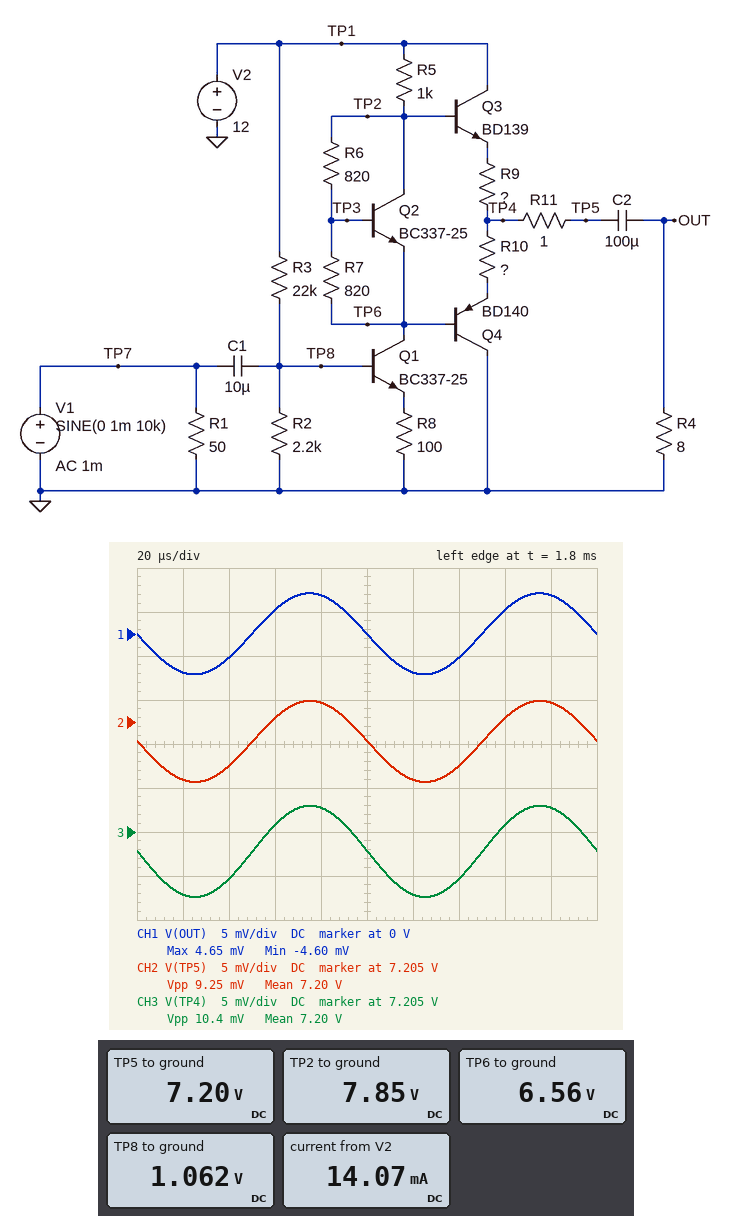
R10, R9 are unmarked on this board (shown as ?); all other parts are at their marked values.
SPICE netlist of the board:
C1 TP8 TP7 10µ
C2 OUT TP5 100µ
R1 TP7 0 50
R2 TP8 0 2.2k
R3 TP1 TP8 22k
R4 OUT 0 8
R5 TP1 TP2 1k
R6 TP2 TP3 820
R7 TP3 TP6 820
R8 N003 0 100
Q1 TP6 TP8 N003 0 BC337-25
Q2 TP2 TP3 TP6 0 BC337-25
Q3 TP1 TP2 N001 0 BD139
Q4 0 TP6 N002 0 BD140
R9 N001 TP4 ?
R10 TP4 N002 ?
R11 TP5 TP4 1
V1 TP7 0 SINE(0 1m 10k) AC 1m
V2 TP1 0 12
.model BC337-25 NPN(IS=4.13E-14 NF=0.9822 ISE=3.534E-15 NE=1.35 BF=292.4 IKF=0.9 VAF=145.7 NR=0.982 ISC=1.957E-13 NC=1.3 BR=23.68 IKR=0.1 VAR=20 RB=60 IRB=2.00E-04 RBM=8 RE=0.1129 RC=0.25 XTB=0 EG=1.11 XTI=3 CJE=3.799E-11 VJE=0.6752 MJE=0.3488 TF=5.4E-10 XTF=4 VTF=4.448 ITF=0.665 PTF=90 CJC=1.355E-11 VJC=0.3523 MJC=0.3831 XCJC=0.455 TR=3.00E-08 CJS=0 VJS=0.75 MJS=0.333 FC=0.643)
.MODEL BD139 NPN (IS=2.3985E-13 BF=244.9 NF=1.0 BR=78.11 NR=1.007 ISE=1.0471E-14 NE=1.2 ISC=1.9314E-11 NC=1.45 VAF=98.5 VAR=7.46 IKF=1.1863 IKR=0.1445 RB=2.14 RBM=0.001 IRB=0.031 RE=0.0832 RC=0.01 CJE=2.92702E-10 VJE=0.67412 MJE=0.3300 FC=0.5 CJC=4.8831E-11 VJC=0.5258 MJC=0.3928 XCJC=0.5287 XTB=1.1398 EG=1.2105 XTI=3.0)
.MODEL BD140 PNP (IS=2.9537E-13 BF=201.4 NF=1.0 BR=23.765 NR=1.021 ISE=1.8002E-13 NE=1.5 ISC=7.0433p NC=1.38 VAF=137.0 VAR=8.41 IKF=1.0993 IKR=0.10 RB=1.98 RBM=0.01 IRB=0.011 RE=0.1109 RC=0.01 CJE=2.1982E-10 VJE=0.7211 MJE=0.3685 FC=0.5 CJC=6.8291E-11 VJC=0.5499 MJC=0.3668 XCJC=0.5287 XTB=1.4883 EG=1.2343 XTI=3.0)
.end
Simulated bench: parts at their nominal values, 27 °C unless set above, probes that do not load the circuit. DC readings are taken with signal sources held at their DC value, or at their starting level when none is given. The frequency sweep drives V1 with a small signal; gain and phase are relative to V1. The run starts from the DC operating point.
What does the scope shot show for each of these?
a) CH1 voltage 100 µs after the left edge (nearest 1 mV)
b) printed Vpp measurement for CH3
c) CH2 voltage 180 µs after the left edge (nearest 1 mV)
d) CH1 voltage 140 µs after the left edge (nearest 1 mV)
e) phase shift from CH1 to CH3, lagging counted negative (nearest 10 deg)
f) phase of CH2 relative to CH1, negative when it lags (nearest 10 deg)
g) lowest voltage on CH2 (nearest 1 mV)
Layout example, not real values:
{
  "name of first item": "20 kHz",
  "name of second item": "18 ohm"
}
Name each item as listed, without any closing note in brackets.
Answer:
{
  "CH1 voltage 100 µs after the left edge": "0 V",
  "printed Vpp measurement for CH3": "10.4 mV",
  "CH2 voltage 180 µs after the left edge": "7.207 V",
  "CH1 voltage 140 µs after the left edge": "-3 mV",
  "phase shift from CH1 to CH3, lagging counted negative": "0 deg",
  "phase of CH2 relative to CH1, negative when it lags": "0 deg",
  "lowest voltage on CH2": "7.198 V"
}
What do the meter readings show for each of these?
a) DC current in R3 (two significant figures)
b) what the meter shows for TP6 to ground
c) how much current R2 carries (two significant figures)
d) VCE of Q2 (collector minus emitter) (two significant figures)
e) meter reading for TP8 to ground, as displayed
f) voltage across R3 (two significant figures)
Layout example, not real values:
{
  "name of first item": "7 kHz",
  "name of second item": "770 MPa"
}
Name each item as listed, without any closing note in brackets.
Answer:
{
  "DC current in R3": "500 µA",
  "what the meter shows for TP6 to ground": "6.56 V",
  "how much current R2 carries": "480 µA",
  "VCE of Q2 (collector minus emitter)": "1.3 V",
  "meter reading for TP8 to ground, as displayed": "1.062 V",
  "voltage across R3": "11 V"
}
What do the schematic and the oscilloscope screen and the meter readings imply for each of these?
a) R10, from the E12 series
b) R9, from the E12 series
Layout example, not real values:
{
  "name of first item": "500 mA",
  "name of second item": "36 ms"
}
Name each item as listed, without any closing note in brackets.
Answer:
{
  "R10, from the E12 series": "1.8 Ω",
  "R9, from the E12 series": "1.2 Ω"
}
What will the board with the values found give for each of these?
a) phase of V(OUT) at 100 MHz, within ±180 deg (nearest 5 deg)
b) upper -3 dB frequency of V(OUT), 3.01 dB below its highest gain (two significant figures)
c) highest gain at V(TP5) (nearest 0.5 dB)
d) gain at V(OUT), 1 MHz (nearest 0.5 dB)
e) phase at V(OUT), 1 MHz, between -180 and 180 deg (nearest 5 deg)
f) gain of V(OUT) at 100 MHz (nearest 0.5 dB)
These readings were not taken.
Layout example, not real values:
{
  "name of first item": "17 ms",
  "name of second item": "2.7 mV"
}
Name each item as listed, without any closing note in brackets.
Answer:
{
  "phase of V(OUT) at 100 MHz, within ±180 deg": "45 deg",
  "upper -3 dB frequency of V(OUT), 3.01 dB below its highest gain": "1.5 MHz",
  "highest gain at V(TP5)": "19.0 dB",
  "gain at V(OUT), 1 MHz": "11.5 dB",
  "phase at V(OUT), 1 MHz, between -180 and 180 deg": "145 deg",
  "gain of V(OUT) at 100 MHz": "-19.5 dB"
}
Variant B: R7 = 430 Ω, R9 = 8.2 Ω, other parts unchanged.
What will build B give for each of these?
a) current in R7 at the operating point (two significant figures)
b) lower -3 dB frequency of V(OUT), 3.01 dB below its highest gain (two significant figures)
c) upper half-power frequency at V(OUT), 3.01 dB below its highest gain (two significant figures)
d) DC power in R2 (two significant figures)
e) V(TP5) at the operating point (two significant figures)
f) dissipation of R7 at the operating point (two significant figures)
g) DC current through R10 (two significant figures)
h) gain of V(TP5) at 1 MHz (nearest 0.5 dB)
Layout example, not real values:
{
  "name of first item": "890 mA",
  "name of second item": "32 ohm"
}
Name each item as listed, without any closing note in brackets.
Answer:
{
  "current in R7 at the operating point": "1.5 mA",
  "lower -3 dB frequency of V(OUT), 3.01 dB below its highest gain": "97 Hz",
  "upper half-power frequency at V(OUT), 3.01 dB below its highest gain": "3.2 MHz",
  "DC power in R2": "510 µW",
  "V(TP5) at the operating point": "6.8 V",
  "dissipation of R7 at the operating point": "930 µW",
  "DC current through R10": "49 mA",
  "gain of V(TP5) at 1 MHz": "13.0 dB"
}
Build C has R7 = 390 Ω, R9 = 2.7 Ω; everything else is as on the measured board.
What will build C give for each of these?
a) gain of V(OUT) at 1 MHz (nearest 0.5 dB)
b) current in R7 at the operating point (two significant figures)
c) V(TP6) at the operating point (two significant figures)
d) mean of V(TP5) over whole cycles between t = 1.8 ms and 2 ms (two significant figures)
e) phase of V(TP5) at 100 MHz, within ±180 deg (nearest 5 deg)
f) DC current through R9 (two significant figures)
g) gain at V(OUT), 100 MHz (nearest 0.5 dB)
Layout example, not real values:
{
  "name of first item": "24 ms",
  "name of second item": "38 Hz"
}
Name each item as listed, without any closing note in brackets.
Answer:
{
  "gain of V(OUT) at 1 MHz": "13.0 dB",
  "current in R7 at the operating point": "1.6 mA",
  "V(TP6) at the operating point": "6.0 V",
  "mean of V(TP5) over whole cycles between t = 1.8 ms and 2 ms": "6.9 V",
  "phase of V(TP5) at 100 MHz, within ±180 deg": "25 deg",
  "DC current through R9": "120 mA",
  "gain at V(OUT), 100 MHz": "-12.5 dB"
}
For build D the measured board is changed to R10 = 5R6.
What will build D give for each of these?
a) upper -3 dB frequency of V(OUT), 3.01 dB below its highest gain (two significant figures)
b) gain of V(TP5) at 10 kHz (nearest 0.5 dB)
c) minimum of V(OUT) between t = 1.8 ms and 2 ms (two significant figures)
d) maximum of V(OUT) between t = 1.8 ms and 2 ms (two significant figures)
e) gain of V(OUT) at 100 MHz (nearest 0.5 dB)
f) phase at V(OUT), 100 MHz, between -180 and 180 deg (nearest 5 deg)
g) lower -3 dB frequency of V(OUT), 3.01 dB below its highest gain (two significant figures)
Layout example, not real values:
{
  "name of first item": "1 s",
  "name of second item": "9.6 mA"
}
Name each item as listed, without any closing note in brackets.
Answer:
{
  "upper -3 dB frequency of V(OUT), 3.01 dB below its highest gain": "1.2 MHz",
  "gain of V(TP5) at 10 kHz": "12.5 dB",
  "minimum of V(OUT) between t = 1.8 ms and 2 ms": "-4.3 mV",
  "maximum of V(OUT) between t = 1.8 ms and 2 ms": "4.3 mV",
  "gain of V(OUT) at 100 MHz": "-21.0 dB",
  "phase at V(OUT), 100 MHz, between -180 and 180 deg": "50 deg",
  "lower -3 dB frequency of V(OUT), 3.01 dB below its highest gain": "92 Hz"
}
